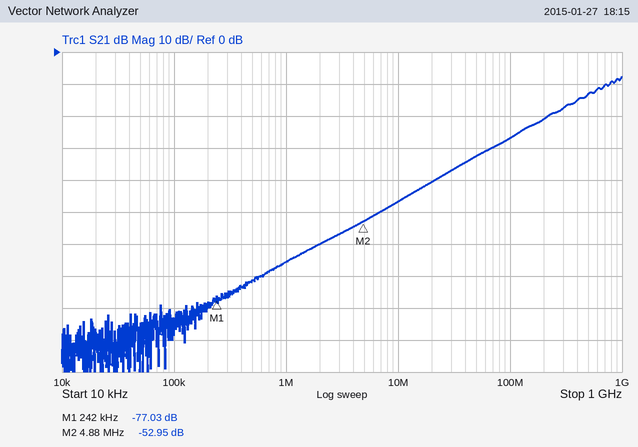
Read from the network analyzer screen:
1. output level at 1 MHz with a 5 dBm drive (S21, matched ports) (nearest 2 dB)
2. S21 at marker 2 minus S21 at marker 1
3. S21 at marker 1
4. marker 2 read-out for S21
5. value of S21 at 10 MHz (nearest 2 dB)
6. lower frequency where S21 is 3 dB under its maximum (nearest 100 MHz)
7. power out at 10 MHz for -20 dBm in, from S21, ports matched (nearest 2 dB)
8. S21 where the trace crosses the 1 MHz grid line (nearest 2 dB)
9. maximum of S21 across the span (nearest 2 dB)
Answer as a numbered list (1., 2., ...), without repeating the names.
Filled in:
1. -60 dBm
2. 24.08 dB
3. -77.03 dB
4. -52.95 dB
5. -46 dB
6. 700 MHz
7. -66 dBm
8. -66 dB
9. -8 dB
